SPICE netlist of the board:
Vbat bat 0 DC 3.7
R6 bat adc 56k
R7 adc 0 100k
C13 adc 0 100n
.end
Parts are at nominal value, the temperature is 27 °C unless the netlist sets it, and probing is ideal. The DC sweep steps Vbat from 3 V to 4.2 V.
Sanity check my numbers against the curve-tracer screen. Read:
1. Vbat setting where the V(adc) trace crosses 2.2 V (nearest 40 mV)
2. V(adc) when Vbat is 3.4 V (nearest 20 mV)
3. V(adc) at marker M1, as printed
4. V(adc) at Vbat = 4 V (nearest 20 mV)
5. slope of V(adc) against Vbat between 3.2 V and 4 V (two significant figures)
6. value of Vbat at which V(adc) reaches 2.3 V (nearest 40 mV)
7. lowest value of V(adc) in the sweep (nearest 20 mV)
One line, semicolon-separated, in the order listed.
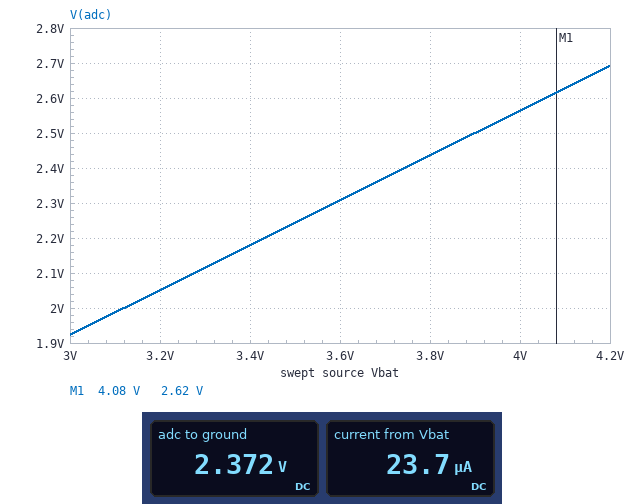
3.44 V; 2.18 V; 2.62 V; 2.56 V; 0.64 V/V; 3.60 V; 1.92 V
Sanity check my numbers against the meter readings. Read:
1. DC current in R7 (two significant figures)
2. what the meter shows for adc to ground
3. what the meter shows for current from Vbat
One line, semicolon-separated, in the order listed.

24 µA; 2.372 V; 23.7 µA
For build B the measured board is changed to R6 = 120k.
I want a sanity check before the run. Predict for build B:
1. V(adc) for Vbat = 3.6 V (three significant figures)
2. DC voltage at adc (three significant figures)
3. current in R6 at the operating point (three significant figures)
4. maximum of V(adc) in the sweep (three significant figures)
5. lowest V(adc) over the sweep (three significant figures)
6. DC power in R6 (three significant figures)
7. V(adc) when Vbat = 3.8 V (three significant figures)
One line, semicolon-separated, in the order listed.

1.64 V; 1.68 V; 16.8 µA; 1.91 V; 1.36 V; 33.9 µW; 1.73 V
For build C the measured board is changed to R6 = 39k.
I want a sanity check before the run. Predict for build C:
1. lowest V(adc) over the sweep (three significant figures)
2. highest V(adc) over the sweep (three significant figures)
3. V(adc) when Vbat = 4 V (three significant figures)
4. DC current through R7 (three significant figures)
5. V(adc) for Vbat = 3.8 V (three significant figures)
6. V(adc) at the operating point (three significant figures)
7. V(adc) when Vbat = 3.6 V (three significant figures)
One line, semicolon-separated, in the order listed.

2.16 V; 3.02 V; 2.88 V; 26.6 µA; 2.73 V; 2.66 V; 2.59 V
